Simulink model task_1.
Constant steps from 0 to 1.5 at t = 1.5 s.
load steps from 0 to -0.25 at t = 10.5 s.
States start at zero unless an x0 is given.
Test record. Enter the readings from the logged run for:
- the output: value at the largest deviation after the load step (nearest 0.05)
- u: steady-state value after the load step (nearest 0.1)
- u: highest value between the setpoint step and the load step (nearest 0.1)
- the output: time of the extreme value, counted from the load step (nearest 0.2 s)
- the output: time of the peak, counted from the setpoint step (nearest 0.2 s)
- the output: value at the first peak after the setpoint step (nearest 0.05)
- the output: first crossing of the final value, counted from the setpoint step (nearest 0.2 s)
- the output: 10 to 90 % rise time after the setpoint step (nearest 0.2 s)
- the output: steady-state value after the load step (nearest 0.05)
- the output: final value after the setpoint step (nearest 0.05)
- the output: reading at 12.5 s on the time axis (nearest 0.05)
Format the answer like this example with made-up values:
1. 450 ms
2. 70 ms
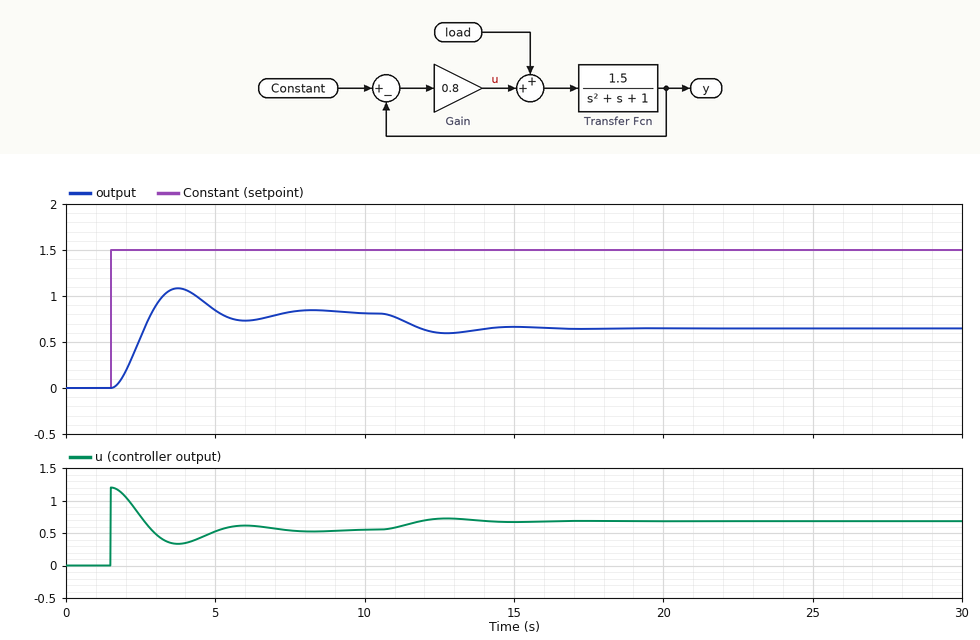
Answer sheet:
1. 0.60
2. 0.7
3. 1.2
4. 2.2 s
5. 2.2 s
6. 1.10
7. 1.4 s
8. 1.0 s
9. 0.65
10. 0.80
11. 0.60
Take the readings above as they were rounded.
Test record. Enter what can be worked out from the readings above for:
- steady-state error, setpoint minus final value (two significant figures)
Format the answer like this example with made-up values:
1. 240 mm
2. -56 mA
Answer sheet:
1. 0.70
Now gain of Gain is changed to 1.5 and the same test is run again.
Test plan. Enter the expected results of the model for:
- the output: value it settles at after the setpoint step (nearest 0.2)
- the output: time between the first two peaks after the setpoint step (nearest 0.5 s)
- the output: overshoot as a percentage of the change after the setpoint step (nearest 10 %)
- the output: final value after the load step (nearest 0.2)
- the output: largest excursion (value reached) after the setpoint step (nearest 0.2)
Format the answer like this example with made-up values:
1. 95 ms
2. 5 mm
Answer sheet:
1. 1.0
2. 3.5 s
3. 40 %
4. 1.0
5. 1.4
